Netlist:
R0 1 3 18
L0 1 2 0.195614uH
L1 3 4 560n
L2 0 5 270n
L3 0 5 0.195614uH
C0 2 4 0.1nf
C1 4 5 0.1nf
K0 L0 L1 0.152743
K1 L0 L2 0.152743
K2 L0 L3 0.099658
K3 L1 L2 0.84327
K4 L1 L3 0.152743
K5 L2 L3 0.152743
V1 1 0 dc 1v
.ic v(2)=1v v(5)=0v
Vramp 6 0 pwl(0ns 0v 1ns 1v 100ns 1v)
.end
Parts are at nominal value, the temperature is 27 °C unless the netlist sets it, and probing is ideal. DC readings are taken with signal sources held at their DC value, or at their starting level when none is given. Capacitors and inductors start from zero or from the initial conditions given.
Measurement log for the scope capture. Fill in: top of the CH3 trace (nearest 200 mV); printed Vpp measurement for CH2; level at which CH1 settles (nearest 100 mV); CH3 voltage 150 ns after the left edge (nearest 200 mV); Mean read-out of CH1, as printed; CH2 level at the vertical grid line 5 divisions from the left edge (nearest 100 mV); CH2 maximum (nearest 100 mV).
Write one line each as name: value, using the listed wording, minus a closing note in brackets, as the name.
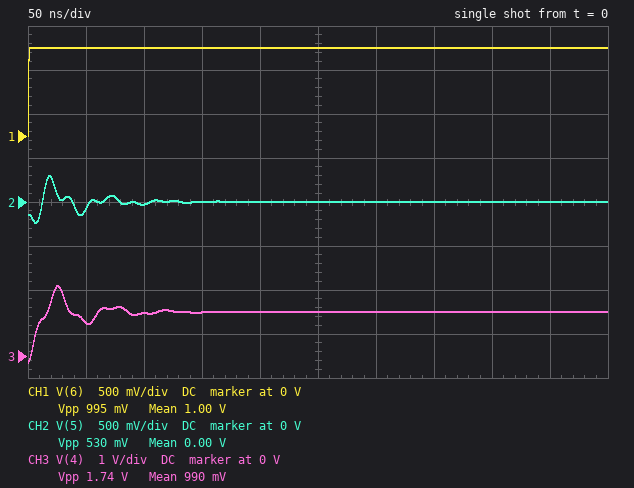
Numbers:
top of the CH3 trace: 1.6 V
printed Vpp measurement for CH2: 530 mV
level at which CH1 settles: 1.0 V
CH3 voltage 150 ns after the left edge: 1.0 V
Mean read-out of CH1, as printed: 1.00 V
CH2 level at the vertical grid line 5 divisions from the left edge: 0 V
CH2 maximum: 300 mV
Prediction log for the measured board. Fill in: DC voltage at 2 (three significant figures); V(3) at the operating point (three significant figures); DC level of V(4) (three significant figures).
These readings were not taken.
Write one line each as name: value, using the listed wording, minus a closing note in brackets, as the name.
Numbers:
DC voltage at 2: 1.00 V
V(3) at the operating point: 1.00 V
DC level of V(4): 1.00 V
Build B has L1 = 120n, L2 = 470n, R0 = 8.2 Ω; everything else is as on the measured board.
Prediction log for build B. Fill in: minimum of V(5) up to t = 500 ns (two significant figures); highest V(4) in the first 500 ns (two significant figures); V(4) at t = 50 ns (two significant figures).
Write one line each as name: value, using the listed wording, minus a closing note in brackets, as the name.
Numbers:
minimum of V(5) up to t = 500 ns: -650 mV
highest V(4) in the first 500 ns: 1.2 V
V(4) at t = 50 ns: 1.1 V
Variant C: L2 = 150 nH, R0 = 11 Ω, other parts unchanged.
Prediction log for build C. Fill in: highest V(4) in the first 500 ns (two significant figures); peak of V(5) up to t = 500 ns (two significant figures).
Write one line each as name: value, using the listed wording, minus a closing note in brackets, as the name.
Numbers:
highest V(4) in the first 500 ns: 1.9 V
peak of V(5) up to t = 500 ns: 220 mV
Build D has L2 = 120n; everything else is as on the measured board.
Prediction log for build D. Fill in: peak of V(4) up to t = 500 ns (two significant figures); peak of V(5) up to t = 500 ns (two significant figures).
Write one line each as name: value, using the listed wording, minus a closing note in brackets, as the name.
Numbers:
peak of V(4) up to t = 500 ns: 1.7 V
peak of V(5) up to t = 500 ns: 190 mV
